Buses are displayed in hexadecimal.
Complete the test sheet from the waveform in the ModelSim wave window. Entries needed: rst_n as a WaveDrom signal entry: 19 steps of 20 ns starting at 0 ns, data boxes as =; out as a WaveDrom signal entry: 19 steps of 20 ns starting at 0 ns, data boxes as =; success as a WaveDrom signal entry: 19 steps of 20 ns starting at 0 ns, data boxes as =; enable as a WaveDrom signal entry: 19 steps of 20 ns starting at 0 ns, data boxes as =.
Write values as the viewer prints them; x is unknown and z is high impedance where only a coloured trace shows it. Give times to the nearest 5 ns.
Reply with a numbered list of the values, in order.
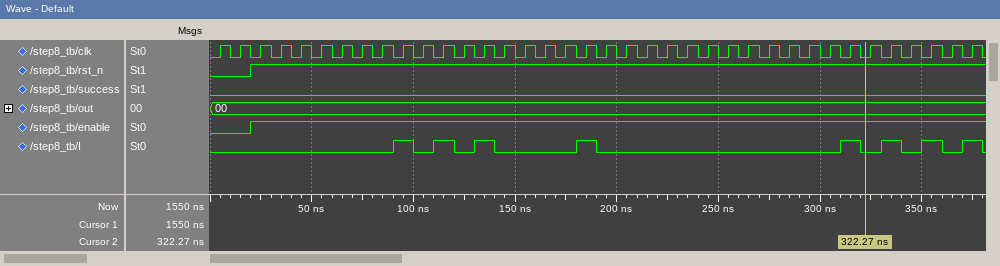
1. {name: 'rst_n', wave: '01.................'}
2. {name: 'out', wave: '=..................', data: '00'}
3. {name: 'success', wave: '0..................'}
4. {name: 'enable', wave: '01.................'}
